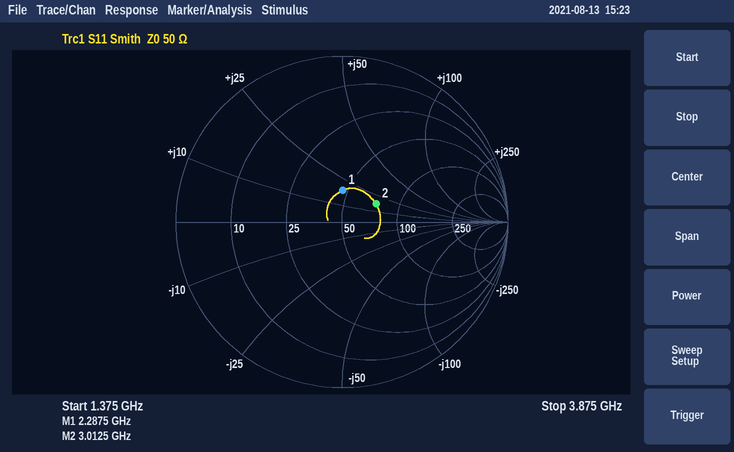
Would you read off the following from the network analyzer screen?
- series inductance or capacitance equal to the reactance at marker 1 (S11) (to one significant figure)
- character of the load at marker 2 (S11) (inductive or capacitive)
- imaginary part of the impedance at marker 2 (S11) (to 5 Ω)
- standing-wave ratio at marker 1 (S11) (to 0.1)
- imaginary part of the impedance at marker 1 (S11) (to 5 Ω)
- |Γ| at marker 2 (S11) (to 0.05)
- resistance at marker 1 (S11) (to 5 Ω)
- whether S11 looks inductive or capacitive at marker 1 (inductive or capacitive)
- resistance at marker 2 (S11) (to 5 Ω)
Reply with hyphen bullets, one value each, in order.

- 1 nH
- inductive
- +15 Ω
- 1.5
- +20 Ω
- 0.25
- 45 Ω
- inductive
- 75 Ω
